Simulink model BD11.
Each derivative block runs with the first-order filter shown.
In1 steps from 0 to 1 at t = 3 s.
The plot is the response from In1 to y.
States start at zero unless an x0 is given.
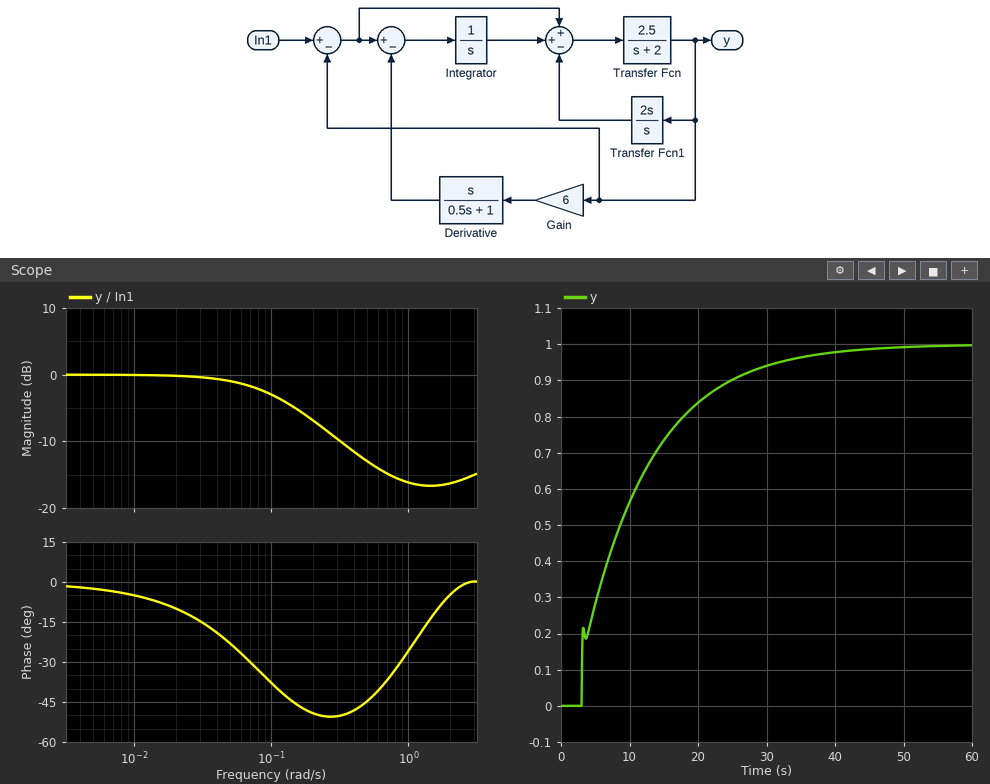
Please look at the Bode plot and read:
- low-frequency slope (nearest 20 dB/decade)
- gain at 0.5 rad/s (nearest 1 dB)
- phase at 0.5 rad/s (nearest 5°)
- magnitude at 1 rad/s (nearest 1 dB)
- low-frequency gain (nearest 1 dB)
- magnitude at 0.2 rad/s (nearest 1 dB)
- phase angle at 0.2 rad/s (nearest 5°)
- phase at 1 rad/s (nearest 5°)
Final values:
0 dB/decade
-13 dB
-45°
-16 dB
0 dB
-7 dB
-50°
-25°
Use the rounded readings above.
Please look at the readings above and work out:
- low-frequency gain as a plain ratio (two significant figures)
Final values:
1.0
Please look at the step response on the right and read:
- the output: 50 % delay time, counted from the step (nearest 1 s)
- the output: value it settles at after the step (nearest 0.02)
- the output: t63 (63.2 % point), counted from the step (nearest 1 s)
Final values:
6 s
1.00
9 s
